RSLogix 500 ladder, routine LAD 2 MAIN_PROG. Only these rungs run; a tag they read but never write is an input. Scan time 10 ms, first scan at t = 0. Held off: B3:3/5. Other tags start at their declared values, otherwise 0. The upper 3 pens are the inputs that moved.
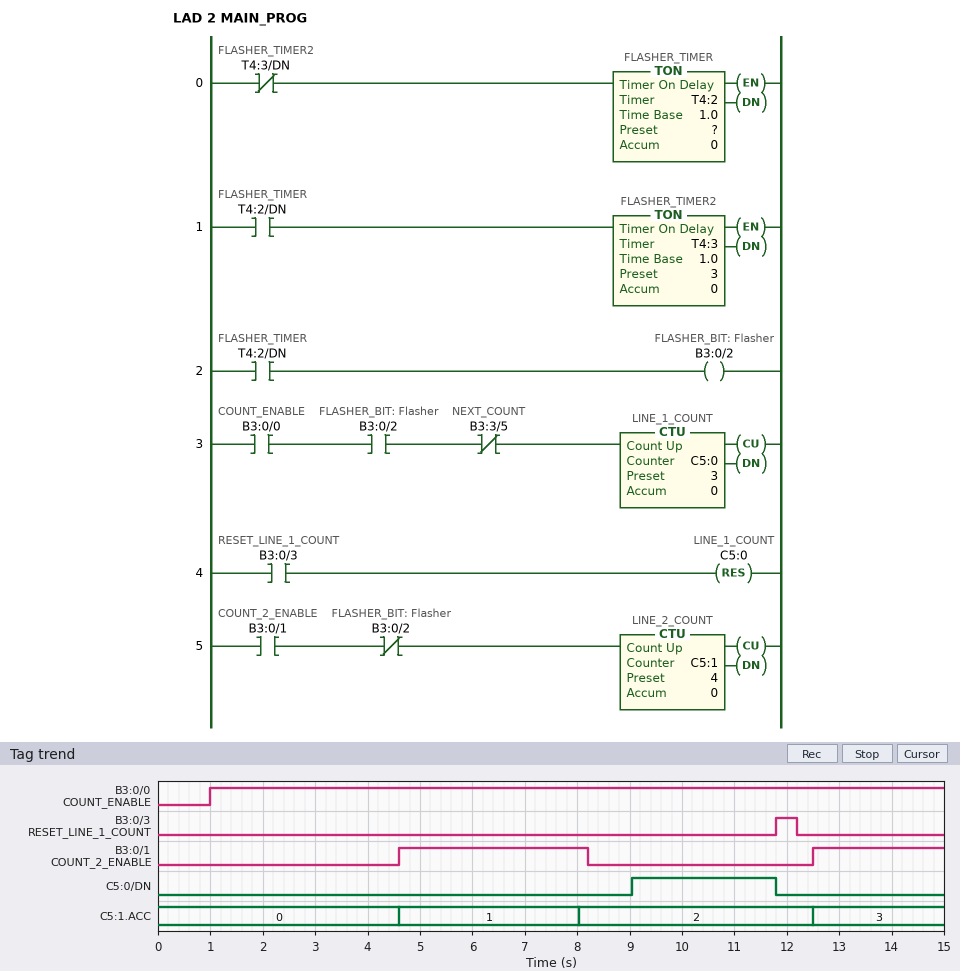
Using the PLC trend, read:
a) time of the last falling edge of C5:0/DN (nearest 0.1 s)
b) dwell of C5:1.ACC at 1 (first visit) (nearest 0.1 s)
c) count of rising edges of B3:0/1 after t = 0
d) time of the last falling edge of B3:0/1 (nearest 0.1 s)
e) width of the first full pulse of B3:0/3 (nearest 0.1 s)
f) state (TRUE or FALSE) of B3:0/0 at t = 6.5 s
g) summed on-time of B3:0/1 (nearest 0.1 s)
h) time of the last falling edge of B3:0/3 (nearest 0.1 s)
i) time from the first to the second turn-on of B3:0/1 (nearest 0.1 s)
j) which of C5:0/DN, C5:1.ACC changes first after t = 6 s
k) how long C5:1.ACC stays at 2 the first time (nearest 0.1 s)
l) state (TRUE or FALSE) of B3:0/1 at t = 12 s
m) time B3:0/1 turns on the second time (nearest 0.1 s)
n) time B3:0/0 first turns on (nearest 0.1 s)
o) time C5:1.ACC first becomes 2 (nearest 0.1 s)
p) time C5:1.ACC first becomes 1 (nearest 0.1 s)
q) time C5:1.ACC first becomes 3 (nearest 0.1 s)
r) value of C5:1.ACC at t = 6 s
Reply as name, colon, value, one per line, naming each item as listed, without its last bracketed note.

time of the last falling edge of C5:0/DN: 11.8 s
dwell of C5:1.ACC at 1 (first visit): 3.4 s
count of rising edges of B3:0/1 after t = 0: 2
time of the last falling edge of B3:0/1: 8.2 s
width of the first full pulse of B3:0/3: 0.4 s
state (TRUE or FALSE) of B3:0/0 at t = 6.5 s: TRUE
summed on-time of B3:0/1: 6.1 s
time of the last falling edge of B3:0/3: 12.2 s
time from the first to the second turn-on of B3:0/1: 7.9 s
which of C5:0/DN, C5:1.ACC changes first after t = 6 s: C5:1.ACC
how long C5:1.ACC stays at 2 the first time: 4.5 s
state (TRUE or FALSE) of B3:0/1 at t = 12 s: FALSE
time B3:0/1 turns on the second time: 12.5 s
time B3:0/0 first turns on: 1.0 s
time C5:1.ACC first becomes 2: 8.0 s
time C5:1.ACC first becomes 1: 4.6 s
time C5:1.ACC first becomes 3: 12.5 s
value of C5:1.ACC at t = 6 s: 1
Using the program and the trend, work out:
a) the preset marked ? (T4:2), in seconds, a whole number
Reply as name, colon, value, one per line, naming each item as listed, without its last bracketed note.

the preset marked ? (T4:2), in seconds, a whole number: 1 s
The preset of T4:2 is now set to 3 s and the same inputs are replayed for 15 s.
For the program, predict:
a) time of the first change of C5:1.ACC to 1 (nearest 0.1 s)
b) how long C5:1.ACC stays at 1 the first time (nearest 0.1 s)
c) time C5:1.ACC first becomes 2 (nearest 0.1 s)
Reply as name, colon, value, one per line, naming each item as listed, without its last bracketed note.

time of the first change of C5:1.ACC to 1: 6.0 s
how long C5:1.ACC stays at 1 the first time: 6.5 s
time C5:1.ACC first becomes 2: 12.5 s
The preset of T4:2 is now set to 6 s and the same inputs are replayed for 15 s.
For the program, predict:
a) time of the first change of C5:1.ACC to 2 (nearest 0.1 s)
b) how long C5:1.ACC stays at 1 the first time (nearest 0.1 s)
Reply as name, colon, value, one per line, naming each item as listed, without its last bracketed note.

time of the first change of C5:1.ACC to 2: 12.5 s
how long C5:1.ACC stays at 1 the first time: 7.9 s
